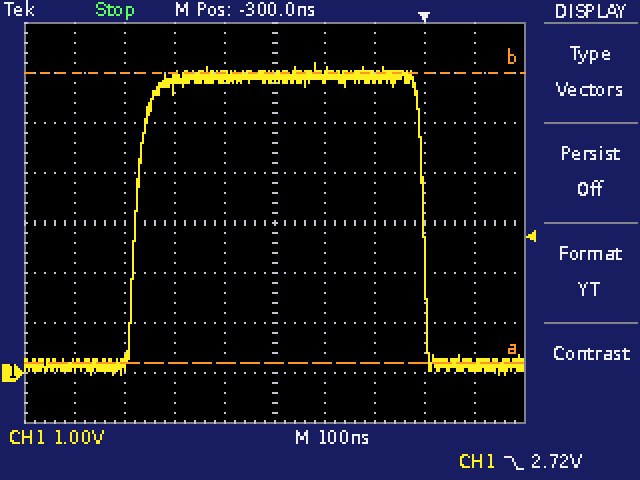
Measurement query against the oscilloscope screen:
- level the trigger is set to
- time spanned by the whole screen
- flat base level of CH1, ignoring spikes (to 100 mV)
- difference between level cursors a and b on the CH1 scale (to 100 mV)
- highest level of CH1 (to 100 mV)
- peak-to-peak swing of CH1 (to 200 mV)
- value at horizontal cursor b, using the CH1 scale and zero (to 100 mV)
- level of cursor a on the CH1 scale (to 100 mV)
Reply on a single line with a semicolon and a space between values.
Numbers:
2.72 V; 1 µs; 200 mV; 5.8 V; 6.2 V; 6.2 V; 6.0 V; 200 mV
